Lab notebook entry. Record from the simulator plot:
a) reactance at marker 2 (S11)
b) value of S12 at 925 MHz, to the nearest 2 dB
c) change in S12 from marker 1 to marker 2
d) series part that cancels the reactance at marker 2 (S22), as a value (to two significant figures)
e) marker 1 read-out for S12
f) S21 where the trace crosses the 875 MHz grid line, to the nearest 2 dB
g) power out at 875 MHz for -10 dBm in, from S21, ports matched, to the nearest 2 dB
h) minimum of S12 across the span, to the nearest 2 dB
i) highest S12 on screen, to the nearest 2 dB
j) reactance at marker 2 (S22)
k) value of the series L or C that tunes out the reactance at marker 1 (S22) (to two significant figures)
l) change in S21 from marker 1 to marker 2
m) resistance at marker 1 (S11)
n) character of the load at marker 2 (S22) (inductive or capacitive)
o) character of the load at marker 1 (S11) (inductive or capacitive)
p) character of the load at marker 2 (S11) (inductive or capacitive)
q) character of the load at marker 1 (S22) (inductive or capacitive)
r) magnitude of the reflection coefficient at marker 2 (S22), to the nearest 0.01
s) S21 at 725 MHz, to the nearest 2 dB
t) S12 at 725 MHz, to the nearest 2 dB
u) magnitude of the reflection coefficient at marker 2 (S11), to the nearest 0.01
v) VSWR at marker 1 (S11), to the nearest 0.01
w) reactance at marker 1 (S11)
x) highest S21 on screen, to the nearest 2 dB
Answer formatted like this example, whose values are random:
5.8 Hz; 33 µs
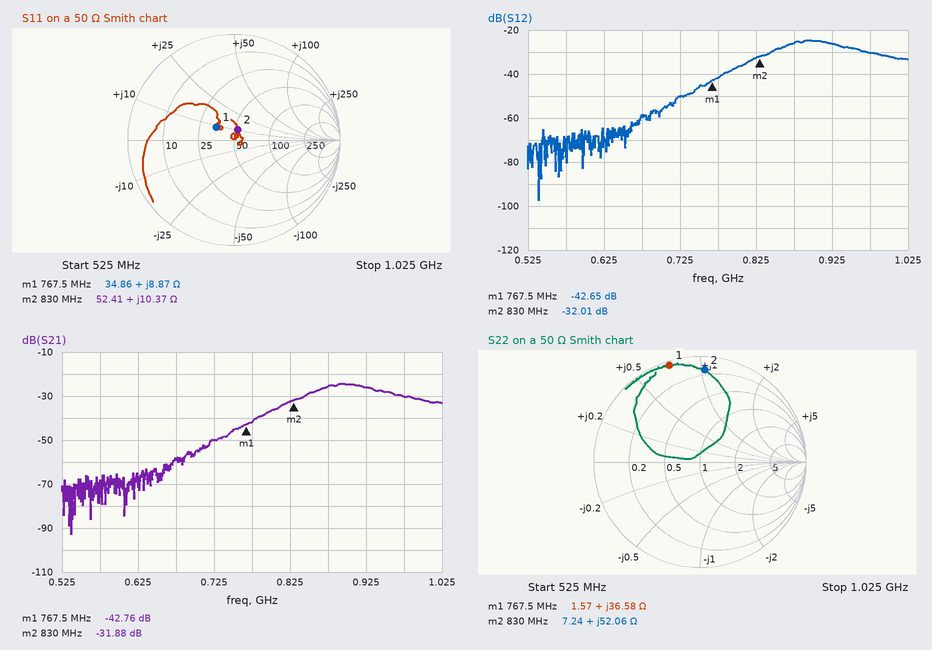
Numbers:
+10.37 Ω; -26 dB; 10.64 dB; 3.7 pF; -42.65 dB; -26 dB; -36 dBm; -98 dB; -24 dB; +52.06 Ω; 5.7 pF; 10.88 dB; 34.86 Ω; inductive; inductive; inductive; inductive; 0.87; -50 dB; -50 dB; 0.10; 1.52; +8.87 Ω; -24 dB
